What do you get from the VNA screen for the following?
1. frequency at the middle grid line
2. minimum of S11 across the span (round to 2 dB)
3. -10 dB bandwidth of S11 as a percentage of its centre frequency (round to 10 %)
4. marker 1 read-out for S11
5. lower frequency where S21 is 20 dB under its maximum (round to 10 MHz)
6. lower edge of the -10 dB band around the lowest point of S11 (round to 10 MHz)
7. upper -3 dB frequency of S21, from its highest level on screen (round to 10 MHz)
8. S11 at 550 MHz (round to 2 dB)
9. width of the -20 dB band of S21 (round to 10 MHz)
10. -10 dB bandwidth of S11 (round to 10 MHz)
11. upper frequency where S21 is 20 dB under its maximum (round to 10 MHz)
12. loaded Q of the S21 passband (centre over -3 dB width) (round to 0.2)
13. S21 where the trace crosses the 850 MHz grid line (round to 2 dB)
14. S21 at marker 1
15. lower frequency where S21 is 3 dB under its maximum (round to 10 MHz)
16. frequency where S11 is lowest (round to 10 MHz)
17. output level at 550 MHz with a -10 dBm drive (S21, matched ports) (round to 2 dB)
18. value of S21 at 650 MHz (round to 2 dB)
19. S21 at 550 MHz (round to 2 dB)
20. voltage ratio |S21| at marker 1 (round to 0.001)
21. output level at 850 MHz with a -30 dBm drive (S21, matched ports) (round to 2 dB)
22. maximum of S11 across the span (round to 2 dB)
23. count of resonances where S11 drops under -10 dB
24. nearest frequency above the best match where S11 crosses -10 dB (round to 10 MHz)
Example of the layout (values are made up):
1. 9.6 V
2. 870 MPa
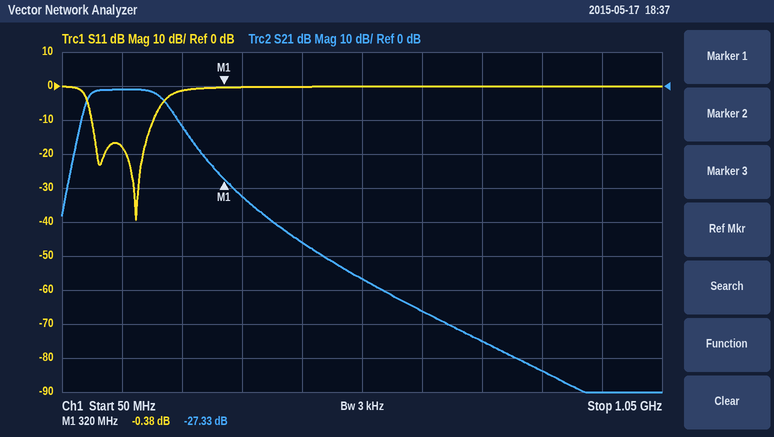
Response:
1. 550 MHz
2. -40 dB
3. 70 %
4. -0.38 dB
5. 70 MHz
6. 100 MHz
7. 220 MHz
8. 0 dB
9. 220 MHz
10. 100 MHz
11. 290 MHz
12. 1.2
13. -84 dB
14. -27.33 dB
15. 90 MHz
16. 170 MHz
17. -66 dBm
18. -66 dB
19. -56 dB
20. 0.043
21. -114 dBm
22. 0 dB
23. 2
24. 200 MHz
